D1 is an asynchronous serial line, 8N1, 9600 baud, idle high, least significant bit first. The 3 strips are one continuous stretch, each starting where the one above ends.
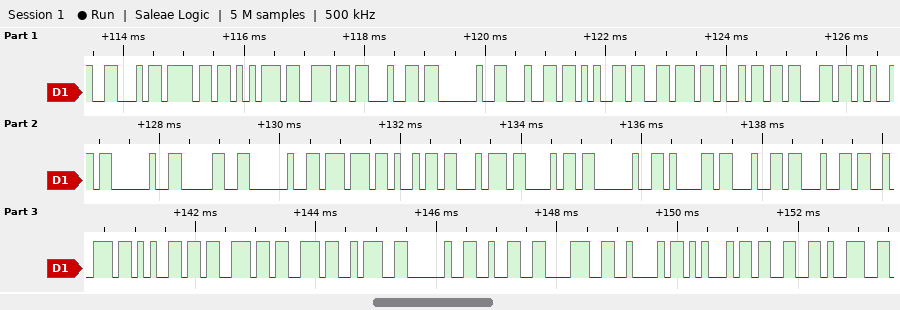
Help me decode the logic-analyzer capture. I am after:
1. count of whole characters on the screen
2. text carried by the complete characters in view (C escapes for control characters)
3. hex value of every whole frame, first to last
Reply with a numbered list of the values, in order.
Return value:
1. 35
2. "Found device 0 with address: 28BE39"
3. 46 6F 75 6E 64 20 64 65 76 69 63 65 20 30 20 77 69 74 68 20 61 64 64 72 65 73 73 3A 20 32 38 42 45 33 39
